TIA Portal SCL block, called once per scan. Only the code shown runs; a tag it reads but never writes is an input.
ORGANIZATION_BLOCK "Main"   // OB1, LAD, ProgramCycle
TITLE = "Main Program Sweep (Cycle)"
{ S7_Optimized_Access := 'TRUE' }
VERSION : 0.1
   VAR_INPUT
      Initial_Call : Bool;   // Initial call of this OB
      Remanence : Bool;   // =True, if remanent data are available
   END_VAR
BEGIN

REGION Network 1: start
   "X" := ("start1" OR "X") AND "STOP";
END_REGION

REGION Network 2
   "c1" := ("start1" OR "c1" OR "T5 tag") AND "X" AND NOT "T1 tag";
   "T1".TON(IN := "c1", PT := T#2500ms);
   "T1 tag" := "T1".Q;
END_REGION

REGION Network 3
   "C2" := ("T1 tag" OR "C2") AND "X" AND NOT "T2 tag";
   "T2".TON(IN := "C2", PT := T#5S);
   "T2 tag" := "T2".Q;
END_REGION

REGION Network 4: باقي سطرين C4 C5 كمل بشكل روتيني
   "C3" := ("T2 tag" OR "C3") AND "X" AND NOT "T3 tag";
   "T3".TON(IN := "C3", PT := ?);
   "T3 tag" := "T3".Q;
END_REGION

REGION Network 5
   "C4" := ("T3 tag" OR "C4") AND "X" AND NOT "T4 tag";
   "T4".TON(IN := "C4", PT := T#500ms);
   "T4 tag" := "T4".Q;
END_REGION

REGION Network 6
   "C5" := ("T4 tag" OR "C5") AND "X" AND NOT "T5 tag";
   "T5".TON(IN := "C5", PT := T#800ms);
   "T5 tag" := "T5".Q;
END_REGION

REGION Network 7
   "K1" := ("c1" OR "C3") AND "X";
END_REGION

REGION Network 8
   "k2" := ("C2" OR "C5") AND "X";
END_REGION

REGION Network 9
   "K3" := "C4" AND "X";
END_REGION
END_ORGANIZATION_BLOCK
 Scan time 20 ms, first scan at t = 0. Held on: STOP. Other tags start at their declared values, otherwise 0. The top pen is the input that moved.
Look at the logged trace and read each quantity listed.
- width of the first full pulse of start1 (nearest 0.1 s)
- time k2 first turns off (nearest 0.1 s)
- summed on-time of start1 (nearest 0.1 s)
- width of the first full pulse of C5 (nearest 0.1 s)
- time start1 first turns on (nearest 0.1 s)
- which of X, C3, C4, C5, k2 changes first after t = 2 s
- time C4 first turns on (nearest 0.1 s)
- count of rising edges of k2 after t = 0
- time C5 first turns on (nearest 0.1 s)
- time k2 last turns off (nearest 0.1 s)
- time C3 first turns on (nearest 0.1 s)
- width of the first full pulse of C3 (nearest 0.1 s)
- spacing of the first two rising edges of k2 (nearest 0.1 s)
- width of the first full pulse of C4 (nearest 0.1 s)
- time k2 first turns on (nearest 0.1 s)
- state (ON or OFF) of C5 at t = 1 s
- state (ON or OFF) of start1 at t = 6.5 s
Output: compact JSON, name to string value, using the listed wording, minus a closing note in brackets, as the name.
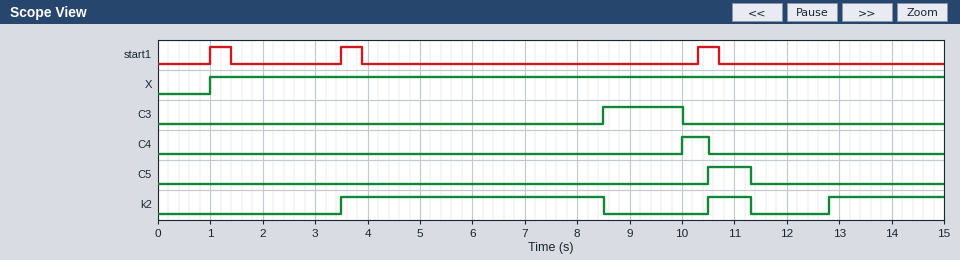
{"width of the first full pulse of start1": "0.4 s", "time k2 first turns off": "8.5 s", "summed on-time of start1": "1.2 s", "width of the first full pulse of C5": "0.8 s", "time start1 first turns on": "1.0 s", "which of X, C3, C4, C5, k2 changes first after t = 2 s": "k2", "time C4 first turns on": "10.0 s", "count of rising edges of k2 after t = 0": "3", "time C5 first turns on": "10.5 s", "time k2 last turns off": "11.3 s", "time C3 first turns on": "8.5 s", "width of the first full pulse of C3": "1.5 s", "spacing of the first two rising edges of k2": "7.0 s", "width of the first full pulse of C4": "0.5 s", "time k2 first turns on": "3.5 s", "state (ON or OFF) of C5 at t = 1 s": "OFF", "state (ON or OFF) of start1 at t = 6.5 s": "OFF"}
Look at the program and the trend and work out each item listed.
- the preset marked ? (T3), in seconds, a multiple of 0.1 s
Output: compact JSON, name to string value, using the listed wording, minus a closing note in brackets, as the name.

{"the preset marked ? (T3), in seconds, a multiple of 0.1 s": "1.5 s"}
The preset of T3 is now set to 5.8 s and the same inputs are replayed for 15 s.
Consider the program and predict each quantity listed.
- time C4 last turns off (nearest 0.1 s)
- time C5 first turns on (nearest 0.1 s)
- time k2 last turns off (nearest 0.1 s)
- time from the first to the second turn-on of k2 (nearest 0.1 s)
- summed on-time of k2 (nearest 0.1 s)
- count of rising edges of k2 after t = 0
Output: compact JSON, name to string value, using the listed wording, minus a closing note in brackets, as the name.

{"time C4 last turns off": "14.8 s", "time C5 first turns on": "14.8 s", "time k2 last turns off": "8.5 s", "time from the first to the second turn-on of k2": "9.3 s", "summed on-time of k2": "7.2 s", "count of rising edges of k2 after t = 0": "2"}
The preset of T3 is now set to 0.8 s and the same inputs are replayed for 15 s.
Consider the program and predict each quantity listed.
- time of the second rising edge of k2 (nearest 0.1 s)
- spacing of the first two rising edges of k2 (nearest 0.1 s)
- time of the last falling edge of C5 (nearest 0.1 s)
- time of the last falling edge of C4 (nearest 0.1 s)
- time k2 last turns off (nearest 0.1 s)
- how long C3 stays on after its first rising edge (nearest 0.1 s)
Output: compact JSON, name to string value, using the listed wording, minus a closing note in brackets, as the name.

{"time of the second rising edge of k2": "9.8 s", "spacing of the first two rising edges of k2": "6.3 s", "time of the last falling edge of C5": "10.6 s", "time of the last falling edge of C4": "9.8 s", "time k2 last turns off": "10.6 s", "how long C3 stays on after its first rising edge": "0.8 s"}
